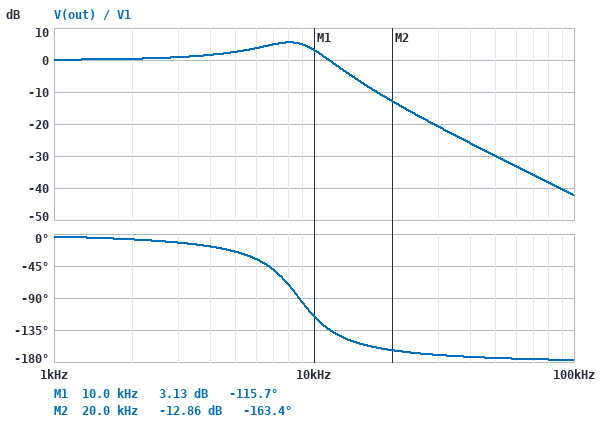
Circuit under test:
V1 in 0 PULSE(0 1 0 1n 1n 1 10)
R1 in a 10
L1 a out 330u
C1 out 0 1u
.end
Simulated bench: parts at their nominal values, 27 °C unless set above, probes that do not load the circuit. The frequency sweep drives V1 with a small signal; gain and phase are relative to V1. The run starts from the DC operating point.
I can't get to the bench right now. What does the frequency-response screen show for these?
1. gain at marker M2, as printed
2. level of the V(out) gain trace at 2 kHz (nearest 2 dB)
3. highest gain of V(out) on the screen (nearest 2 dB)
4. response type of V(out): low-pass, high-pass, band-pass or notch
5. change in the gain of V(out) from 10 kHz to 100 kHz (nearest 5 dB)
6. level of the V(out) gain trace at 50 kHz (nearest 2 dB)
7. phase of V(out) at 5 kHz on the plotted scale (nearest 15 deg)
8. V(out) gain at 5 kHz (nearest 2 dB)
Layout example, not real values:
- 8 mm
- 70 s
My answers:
- -12.86 dB
- 0 dB
- 6 dB
- low-pass
- -45 dB
- -30 dB
- -30 deg
- 2 dB
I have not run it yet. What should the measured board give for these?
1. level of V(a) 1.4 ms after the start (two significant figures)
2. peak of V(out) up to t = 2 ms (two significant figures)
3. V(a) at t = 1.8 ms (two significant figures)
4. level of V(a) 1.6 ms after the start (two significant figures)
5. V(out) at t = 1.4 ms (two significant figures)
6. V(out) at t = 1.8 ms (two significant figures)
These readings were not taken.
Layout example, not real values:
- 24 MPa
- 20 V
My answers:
- 1.0 V
- 1.4 V
- 1.0 V
- 1.0 V
- 1.0 V
- 1.0 V
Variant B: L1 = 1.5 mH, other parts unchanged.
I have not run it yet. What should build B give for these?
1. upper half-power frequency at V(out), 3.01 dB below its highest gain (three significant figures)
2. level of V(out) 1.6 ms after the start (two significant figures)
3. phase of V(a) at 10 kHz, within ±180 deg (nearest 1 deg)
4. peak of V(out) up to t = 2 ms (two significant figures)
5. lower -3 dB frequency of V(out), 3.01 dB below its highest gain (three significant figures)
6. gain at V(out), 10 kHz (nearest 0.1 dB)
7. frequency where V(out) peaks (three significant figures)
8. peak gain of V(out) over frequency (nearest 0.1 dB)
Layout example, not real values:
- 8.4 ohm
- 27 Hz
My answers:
- 4.54 kHz
- 1.0 V
- 7 deg
- 1.7 V
- 3.46 kHz
- -13.9 dB
- 4.04 kHz
- 11.8 dB
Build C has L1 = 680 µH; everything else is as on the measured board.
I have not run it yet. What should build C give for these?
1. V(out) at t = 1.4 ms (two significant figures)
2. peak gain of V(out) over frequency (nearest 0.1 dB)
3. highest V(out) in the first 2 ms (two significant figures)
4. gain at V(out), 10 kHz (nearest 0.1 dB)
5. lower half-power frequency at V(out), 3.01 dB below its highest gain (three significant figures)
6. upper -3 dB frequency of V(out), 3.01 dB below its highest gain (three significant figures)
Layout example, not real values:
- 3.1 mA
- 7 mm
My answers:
- 1.0 V
- 8.5 dB
- 1.5 V
- -5.1 dB
- 4.53 kHz
- 6.97 kHz
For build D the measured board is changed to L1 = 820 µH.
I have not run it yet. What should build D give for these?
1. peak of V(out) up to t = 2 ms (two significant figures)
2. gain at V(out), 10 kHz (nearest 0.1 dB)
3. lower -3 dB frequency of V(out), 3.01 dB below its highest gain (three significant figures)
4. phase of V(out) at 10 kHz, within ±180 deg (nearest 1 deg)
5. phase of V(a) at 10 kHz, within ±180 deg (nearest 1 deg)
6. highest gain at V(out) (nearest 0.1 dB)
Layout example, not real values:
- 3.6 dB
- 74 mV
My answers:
- 1.6 V
- -7.3 dB
- 4.29 kHz
- -164 deg
- 16 deg
- 9.3 dB
